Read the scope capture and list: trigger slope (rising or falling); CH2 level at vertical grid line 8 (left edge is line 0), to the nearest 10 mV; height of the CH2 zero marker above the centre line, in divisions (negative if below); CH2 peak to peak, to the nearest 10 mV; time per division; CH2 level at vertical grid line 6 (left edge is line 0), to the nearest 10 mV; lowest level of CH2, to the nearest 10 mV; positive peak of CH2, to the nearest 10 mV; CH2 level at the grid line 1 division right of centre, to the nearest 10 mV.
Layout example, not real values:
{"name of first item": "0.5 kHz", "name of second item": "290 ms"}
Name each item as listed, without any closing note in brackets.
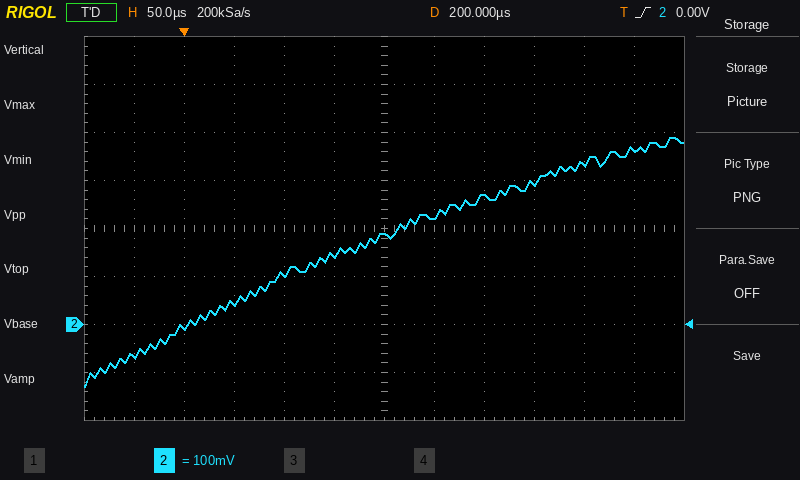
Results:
{"trigger slope": "rising", "CH2 level at vertical grid line 8 (left edge is line 0), to the nearest 10 mV": "270 mV", "height of the CH2 zero marker above the centre line, in divisions": "-2.0 div", "CH2 peak to peak, to the nearest 10 mV": "520 mV", "time per division": "50 µs", "CH2 level at vertical grid line 6 (left edge is line 0), to the nearest 10 mV": "190 mV", "lowest level of CH2, to the nearest 10 mV": "-130 mV", "positive peak of CH2, to the nearest 10 mV": "390 mV", "CH2 level at the grid line 1 division right of centre, to the nearest 10 mV": "220 mV"}
